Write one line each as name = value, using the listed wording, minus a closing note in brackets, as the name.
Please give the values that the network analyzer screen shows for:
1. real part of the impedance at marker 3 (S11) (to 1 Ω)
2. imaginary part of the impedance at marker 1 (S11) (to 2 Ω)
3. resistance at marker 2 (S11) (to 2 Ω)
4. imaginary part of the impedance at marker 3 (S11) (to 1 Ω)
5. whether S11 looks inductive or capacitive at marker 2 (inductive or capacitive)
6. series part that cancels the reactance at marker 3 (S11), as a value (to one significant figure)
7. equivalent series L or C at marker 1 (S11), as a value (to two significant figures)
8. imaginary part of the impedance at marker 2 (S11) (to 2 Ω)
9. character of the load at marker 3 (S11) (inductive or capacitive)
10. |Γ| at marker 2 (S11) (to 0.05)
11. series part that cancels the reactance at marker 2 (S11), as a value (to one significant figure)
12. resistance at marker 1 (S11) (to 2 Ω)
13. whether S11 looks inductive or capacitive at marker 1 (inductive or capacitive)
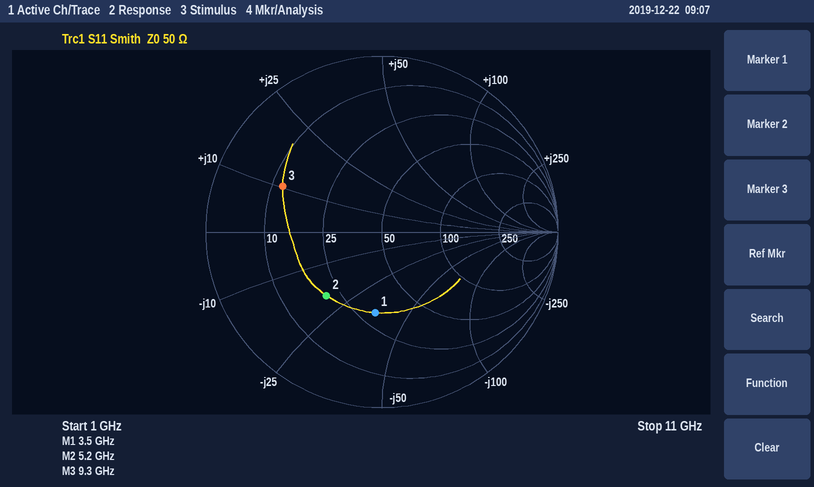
real part of the impedance at marker 3 (S11) = 12 Ω
imaginary part of the impedance at marker 1 (S11) = -36 Ω
resistance at marker 2 (S11) = 20 Ω
imaginary part of the impedance at marker 3 (S11) = +10 Ω
whether S11 looks inductive or capacitive at marker 2 = capacitive
series part that cancels the reactance at marker 3 (S11), as a value = 2 pF
equivalent series L or C at marker 1 (S11), as a value = 1.3 pF
imaginary part of the impedance at marker 2 (S11) = -20 Ω
character of the load at marker 3 (S11) = inductive
|Γ| at marker 2 (S11) = 0.50
series part that cancels the reactance at marker 2 (S11), as a value = 600 pH
resistance at marker 1 (S11) = 30 Ω
whether S11 looks inductive or capacitive at marker 1 = capacitive
